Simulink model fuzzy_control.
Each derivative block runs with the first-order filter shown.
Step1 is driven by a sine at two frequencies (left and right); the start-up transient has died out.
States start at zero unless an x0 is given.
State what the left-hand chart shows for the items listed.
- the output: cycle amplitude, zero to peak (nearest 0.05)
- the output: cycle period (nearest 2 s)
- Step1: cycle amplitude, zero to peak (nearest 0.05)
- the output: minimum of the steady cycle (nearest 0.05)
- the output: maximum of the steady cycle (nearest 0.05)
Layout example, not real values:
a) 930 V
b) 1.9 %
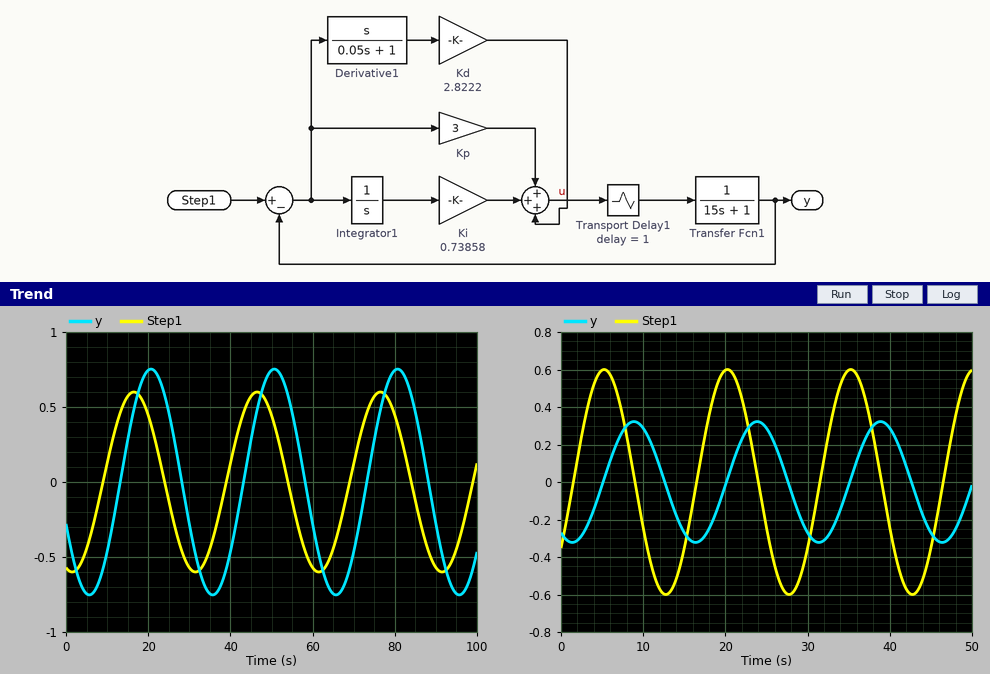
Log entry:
a) 0.75
b) 30 s
c) 0.60
d) -0.75
e) 0.75
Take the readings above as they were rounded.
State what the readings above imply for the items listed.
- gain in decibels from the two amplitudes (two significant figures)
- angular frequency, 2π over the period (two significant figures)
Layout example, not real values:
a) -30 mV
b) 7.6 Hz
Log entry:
a) 1.9 dB
b) 0.21 rad/s
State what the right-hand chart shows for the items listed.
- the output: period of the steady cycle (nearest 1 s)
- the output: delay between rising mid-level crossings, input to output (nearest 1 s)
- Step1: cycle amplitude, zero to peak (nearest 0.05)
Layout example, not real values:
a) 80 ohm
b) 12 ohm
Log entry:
a) 15 s
b) 4 s
c) 0.60
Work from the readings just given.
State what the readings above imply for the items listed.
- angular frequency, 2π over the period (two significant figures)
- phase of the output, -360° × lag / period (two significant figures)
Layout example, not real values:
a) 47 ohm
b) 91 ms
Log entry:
a) 0.42 rad/s
b) -96°
